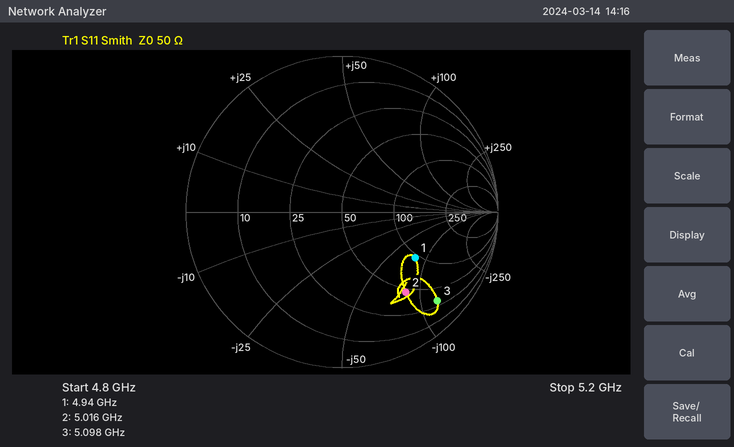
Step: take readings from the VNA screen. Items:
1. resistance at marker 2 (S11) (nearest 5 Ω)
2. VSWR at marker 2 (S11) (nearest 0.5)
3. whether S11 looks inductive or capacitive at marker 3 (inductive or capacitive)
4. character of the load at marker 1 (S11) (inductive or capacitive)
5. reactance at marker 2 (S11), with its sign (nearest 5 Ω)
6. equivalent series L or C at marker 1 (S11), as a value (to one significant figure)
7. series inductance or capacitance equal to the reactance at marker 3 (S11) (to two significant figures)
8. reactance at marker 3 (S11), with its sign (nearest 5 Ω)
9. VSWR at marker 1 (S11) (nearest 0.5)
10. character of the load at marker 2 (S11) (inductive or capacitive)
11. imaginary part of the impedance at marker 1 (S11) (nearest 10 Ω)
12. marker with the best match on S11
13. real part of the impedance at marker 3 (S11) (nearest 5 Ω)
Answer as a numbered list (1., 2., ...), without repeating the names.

1. 45 Ω
2. 5.0
3. capacitive
4. capacitive
5. -85 Ω
6. 400 fF
7. 260 fF
8. -120 Ω
9. 3.5
10. capacitive
11. -80 Ω
12. marker 1
13. 30 Ω
